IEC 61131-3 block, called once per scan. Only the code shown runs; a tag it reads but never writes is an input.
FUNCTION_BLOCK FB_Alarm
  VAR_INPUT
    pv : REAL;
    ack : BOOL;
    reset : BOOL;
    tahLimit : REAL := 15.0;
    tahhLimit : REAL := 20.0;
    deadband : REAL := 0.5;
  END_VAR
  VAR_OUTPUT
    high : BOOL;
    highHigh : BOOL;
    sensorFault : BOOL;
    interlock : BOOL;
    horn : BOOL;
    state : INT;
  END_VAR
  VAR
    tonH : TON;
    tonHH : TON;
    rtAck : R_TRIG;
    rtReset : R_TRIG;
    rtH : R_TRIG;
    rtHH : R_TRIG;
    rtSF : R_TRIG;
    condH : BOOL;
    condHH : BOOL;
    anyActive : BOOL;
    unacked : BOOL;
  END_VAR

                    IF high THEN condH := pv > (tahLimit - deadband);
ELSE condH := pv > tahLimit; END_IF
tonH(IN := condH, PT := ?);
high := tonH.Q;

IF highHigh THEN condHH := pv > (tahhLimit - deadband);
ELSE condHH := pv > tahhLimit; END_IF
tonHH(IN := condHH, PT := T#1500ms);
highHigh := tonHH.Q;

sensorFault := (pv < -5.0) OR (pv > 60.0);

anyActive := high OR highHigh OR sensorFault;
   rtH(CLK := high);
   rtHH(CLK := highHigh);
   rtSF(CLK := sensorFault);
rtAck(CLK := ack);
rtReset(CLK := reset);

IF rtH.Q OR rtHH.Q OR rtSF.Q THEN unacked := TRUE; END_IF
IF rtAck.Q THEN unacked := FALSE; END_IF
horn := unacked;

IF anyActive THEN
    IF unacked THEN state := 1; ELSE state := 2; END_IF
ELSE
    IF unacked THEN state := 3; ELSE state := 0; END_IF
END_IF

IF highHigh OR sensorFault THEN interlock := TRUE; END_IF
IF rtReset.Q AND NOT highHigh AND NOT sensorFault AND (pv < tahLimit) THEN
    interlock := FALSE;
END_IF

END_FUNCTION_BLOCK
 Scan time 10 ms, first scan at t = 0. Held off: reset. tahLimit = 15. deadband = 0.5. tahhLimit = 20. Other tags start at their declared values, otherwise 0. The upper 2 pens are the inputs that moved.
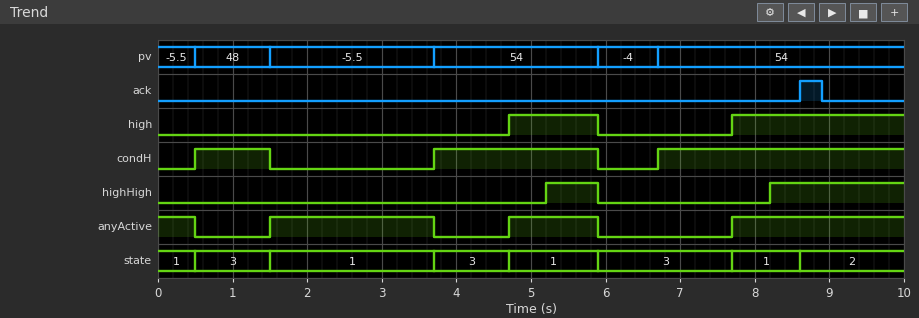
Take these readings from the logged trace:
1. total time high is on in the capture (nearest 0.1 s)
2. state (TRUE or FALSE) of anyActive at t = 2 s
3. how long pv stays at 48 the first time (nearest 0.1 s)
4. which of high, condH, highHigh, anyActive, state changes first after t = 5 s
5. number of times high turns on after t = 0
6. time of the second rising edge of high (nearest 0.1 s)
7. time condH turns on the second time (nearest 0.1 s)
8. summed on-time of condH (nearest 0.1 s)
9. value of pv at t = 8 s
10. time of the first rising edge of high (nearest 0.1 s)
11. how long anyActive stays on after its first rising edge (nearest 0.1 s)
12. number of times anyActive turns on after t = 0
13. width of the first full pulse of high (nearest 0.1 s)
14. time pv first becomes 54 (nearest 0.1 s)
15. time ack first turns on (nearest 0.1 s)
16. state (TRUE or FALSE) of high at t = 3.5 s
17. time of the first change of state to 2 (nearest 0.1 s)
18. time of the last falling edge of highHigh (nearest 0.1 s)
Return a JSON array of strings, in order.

["3.5 s", "TRUE", "1.0 s", "highHigh", "2", "7.7 s", "3.7 s", "6.5 s", "54", "4.7 s", "2.2 s", "3", "1.2 s", "3.7 s", "8.6 s", "FALSE", "8.6 s", "5.9 s"]
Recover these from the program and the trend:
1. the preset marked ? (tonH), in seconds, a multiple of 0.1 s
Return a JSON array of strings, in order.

["1.0 s"]
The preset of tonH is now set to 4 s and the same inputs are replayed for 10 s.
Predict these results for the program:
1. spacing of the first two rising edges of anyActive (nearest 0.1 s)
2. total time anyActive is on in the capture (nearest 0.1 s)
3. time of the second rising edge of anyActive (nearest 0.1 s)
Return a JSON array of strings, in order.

["3.7 s", "5.2 s", "5.2 s"]
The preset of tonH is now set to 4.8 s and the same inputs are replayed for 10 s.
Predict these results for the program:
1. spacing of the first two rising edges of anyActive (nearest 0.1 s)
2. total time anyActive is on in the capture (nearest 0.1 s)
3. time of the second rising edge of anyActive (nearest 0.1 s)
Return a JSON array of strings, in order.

["3.7 s", "5.2 s", "5.2 s"]
